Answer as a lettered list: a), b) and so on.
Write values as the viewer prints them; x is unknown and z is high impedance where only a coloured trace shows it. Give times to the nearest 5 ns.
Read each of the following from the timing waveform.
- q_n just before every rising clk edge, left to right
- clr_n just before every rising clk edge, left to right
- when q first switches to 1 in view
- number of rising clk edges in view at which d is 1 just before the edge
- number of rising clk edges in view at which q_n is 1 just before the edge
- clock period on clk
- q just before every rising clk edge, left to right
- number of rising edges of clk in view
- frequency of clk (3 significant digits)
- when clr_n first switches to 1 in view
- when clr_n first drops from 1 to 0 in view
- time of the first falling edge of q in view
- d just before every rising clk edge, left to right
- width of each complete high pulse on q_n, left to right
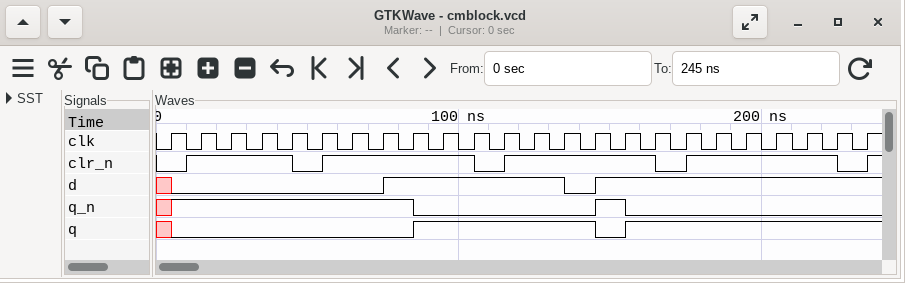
a) x 1 1 1 1 1 1 1 1 0 0 0 0 0 0 1 0 0 0 0 0 0 0 0
b) 0 1 1 1 1 0 1 1 1 1 1 0 1 1 1 1 1 0 1 1 1 1 1 0
c) 85 ns
d) 15
e) 9
f) 10 ns
g) x 0 0 0 0 0 0 0 0 1 1 1 1 1 1 0 1 1 1 1 1 1 1 1
h) 24
i) 100 MHz
j) 10 ns
k) 45 ns
l) 145 ns
m) x 0 0 0 0 0 0 0 1 1 1 1 1 1 0 1 1 1 1 1 1 1 1 1
n) 10 ns
